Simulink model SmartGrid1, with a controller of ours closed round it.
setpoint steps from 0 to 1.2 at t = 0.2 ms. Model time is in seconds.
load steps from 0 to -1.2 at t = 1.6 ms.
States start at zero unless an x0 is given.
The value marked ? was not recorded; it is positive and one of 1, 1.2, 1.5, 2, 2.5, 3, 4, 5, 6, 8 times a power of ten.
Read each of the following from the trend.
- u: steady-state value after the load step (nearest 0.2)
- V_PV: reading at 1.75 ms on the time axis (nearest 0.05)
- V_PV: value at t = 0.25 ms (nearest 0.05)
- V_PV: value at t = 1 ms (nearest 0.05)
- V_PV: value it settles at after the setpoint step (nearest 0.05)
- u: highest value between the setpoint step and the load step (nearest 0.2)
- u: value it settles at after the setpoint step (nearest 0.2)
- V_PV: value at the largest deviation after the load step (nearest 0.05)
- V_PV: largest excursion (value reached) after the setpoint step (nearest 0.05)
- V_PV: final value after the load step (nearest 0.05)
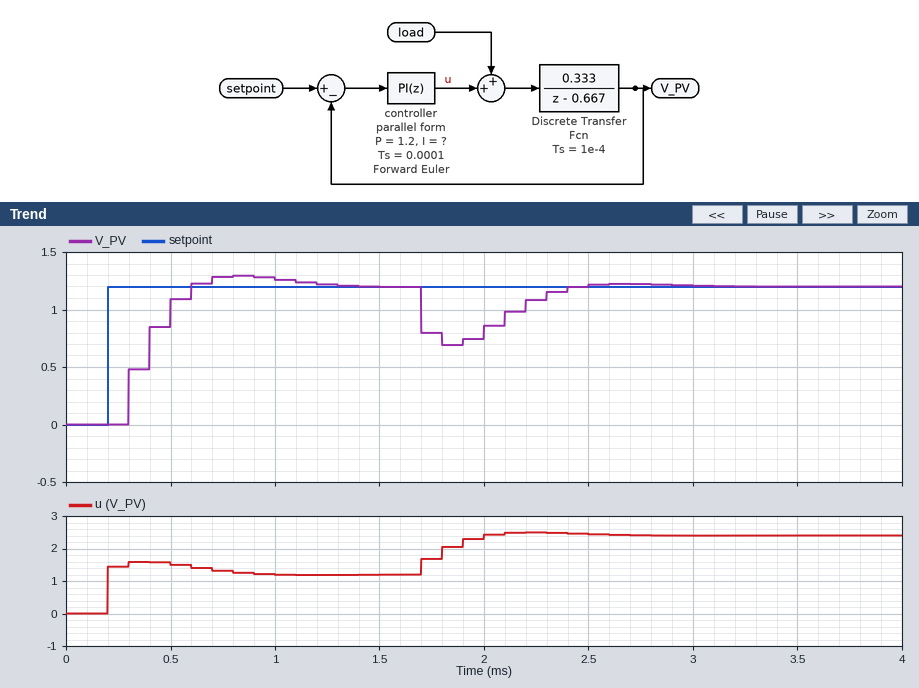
2.4
0.80
0.00
1.25
1.20
1.6
1.2
0.70
1.30
1.20
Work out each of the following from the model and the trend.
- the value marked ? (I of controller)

6000
